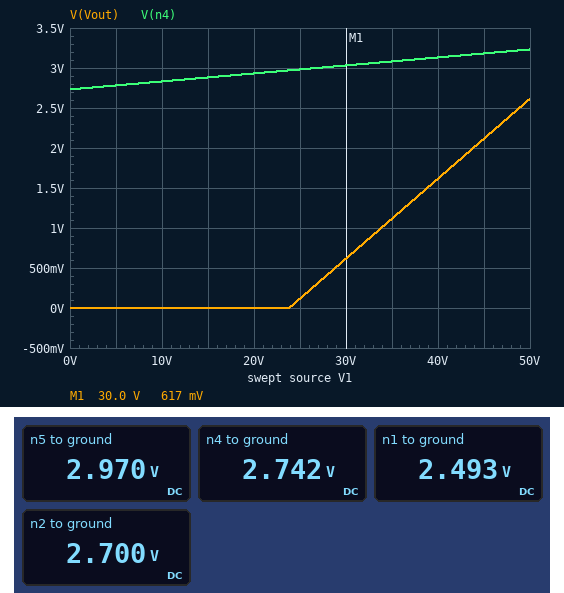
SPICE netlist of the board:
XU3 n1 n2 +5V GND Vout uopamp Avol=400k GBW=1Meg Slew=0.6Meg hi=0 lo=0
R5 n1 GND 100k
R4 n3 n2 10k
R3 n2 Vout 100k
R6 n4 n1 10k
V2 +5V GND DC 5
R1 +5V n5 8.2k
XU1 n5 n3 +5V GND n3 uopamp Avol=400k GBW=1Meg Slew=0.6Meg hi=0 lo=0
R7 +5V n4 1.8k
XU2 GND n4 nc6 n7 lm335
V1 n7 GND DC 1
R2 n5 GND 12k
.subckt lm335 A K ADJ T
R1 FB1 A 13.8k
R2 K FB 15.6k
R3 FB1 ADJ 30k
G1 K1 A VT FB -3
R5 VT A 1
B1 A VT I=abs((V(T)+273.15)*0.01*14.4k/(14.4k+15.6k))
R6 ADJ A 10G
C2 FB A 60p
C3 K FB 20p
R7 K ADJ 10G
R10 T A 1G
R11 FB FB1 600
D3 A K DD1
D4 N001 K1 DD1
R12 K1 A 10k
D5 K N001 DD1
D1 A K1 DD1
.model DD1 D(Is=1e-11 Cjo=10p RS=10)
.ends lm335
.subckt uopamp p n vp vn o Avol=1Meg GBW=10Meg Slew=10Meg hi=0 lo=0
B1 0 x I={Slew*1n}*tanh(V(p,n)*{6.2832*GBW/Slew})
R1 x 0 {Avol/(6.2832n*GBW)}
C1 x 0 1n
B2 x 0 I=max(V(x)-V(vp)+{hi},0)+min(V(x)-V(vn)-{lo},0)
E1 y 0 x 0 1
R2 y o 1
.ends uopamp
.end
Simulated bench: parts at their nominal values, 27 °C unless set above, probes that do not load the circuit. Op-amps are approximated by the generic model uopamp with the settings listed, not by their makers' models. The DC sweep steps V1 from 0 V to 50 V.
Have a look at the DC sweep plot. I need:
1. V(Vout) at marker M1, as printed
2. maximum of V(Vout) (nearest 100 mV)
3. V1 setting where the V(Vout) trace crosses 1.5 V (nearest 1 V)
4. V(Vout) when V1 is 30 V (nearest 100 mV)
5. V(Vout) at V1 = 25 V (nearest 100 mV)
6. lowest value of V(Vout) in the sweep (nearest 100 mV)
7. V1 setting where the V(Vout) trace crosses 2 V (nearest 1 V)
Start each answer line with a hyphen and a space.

- 617 mV
- 2.6 V
- 39 V
- 600 mV
- 100 mV
- 0 V
- 44 V
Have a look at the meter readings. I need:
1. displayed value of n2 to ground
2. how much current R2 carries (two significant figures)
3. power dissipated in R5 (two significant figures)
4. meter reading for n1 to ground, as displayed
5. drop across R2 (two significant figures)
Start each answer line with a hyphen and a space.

- 2.700 V
- 250 µA
- 62 µW
- 2.493 V
- 3.0 V
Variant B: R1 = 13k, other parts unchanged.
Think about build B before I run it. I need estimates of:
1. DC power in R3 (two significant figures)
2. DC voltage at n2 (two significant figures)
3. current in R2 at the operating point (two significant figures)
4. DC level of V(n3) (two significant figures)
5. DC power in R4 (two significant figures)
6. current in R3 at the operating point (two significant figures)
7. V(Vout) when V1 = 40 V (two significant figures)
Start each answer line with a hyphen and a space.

- 8.6 µW
- 2.5 V
- 200 µA
- 2.4 V
- 860 nW
- 9.3 µA
- 5.0 V
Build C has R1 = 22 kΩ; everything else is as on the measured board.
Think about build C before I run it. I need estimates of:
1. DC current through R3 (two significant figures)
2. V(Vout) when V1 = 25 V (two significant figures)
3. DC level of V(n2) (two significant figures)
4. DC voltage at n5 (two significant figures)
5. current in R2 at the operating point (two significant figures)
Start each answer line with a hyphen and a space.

- 29 µA
- 5.0 V
- 2.1 V
- 1.8 V
- 150 µA
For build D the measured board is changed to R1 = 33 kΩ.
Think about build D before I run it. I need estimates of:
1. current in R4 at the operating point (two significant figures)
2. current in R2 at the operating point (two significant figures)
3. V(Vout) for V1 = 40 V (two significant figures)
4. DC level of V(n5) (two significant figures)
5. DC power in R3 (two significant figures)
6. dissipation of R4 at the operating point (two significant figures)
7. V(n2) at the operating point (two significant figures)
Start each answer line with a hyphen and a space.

- 33 µA
- 110 µA
- 5.0 V
- 1.3 V
- 110 µW
- 11 µW
- 1.7 V
